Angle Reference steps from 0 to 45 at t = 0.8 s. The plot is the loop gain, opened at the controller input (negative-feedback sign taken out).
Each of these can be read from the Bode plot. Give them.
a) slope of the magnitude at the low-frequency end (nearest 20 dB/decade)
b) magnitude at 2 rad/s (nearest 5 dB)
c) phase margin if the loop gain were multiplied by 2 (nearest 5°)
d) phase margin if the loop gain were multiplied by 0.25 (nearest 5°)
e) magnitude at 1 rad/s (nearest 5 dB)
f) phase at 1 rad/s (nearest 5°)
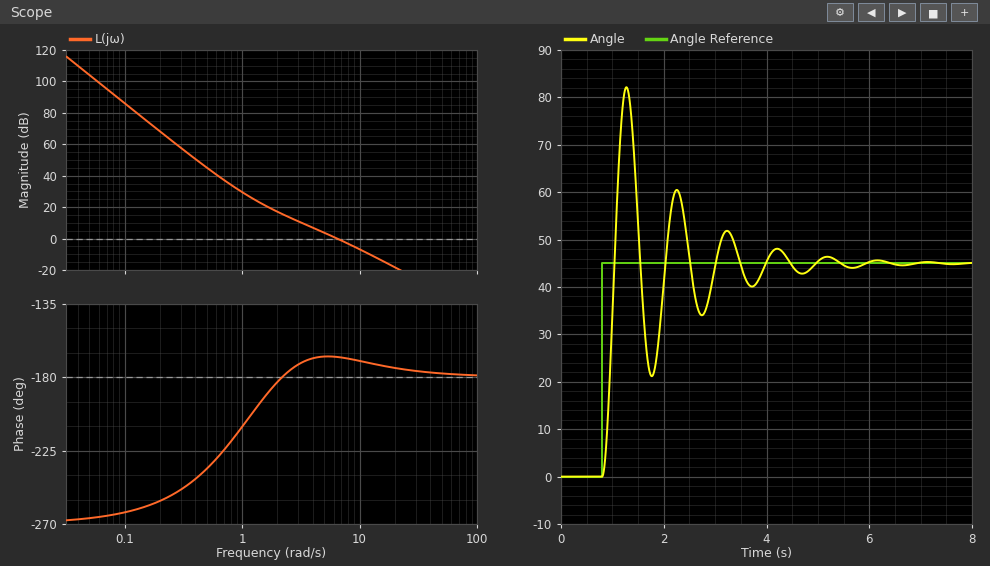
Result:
-60 dB/decade
15 dB
10°
5°
30 dB
-210°
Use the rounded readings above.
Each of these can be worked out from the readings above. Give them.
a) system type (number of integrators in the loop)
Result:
3
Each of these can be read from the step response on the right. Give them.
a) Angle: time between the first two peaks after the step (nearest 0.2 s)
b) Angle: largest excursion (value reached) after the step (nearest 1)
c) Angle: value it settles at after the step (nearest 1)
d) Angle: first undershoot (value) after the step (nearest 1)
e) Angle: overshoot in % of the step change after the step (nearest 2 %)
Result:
1.0 s
82
45
21
82 %
